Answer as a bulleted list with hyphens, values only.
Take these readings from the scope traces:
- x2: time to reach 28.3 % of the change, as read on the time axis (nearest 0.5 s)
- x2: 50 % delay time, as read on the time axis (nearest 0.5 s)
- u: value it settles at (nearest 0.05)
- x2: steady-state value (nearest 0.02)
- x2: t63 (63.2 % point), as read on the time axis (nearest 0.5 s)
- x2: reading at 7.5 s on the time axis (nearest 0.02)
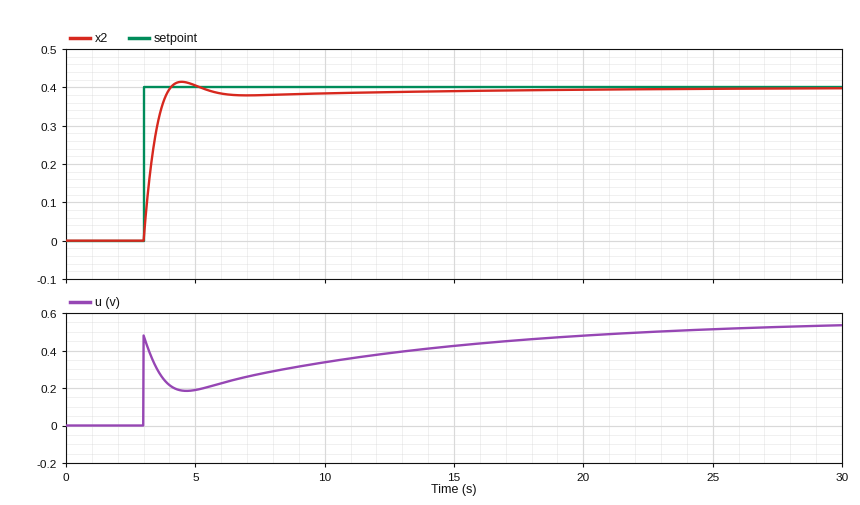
- 3.0 s
- 3.5 s
- 0.55
- 0.40
- 3.5 s
- 0.38
